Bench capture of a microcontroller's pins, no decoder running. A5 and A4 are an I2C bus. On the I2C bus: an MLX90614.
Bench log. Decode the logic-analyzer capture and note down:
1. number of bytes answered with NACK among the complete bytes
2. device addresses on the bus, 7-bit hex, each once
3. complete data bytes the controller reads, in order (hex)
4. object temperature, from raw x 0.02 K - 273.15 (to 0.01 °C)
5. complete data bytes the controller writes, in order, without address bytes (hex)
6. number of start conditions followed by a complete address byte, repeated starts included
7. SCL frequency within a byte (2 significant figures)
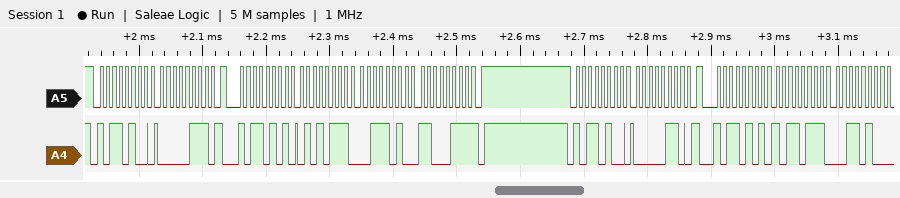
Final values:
1
0x5A
57 3A C7 B7 34
25.55 °C
07 06
4
100 kHz
